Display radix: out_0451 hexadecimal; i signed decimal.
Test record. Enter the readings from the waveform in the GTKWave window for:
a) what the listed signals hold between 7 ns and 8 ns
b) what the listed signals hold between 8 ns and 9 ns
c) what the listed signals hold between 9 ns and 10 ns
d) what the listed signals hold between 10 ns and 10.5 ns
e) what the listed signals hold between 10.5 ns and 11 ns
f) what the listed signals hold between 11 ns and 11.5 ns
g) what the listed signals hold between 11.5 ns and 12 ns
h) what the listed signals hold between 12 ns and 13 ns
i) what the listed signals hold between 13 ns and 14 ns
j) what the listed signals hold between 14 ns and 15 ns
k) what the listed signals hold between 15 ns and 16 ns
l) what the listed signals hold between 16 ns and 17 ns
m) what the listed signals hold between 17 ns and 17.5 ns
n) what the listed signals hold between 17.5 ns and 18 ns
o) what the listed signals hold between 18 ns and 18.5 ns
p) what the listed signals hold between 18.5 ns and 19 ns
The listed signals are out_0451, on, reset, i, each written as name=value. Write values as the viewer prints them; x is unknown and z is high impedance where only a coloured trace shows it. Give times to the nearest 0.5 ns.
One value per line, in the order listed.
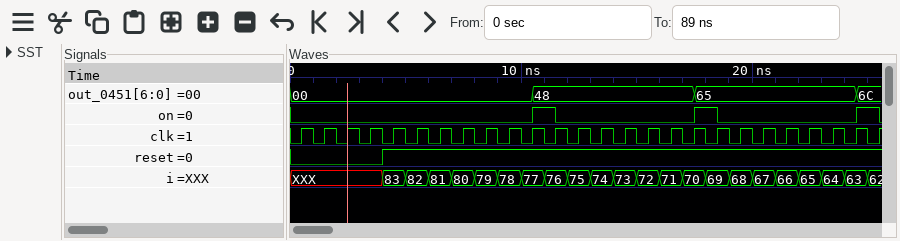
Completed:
out_0451=00, on=0, reset=1, i=80
out_0451=00, on=0, reset=1, i=79
out_0451=00, on=0, reset=1, i=78
out_0451=00, on=0, reset=1, i=77
out_0451=48, on=1, reset=1, i=77
out_0451=48, on=1, reset=1, i=76
out_0451=48, on=0, reset=1, i=76
out_0451=48, on=0, reset=1, i=75
out_0451=48, on=0, reset=1, i=74
out_0451=48, on=0, reset=1, i=73
out_0451=48, on=0, reset=1, i=72
out_0451=48, on=0, reset=1, i=71
out_0451=48, on=0, reset=1, i=70
out_0451=65, on=1, reset=1, i=70
out_0451=65, on=1, reset=1, i=69
out_0451=65, on=0, reset=1, i=69
